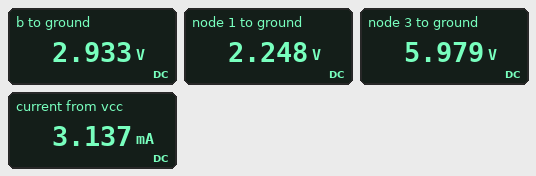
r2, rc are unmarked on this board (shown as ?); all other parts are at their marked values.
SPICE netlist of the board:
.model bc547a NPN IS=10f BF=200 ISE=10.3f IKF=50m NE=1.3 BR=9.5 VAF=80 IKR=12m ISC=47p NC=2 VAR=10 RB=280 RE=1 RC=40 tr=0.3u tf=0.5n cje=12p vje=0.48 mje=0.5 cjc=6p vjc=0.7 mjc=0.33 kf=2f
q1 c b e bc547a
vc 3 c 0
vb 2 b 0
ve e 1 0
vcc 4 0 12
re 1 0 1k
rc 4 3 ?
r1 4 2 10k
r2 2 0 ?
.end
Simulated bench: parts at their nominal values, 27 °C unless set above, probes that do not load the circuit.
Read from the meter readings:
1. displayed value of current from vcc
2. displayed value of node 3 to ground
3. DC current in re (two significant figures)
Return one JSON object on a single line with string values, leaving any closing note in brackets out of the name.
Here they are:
{"displayed value of current from vcc": "3.137 mA", "displayed value of node 3 to ground": "5.979 V", "DC current in re": "2.2 mA"}
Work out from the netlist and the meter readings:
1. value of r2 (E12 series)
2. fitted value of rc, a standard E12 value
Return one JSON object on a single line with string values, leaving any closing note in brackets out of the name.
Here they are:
{"value of r2": "3.3 kΩ", "fitted value of rc, a standard E12 value": "2.7 kΩ"}
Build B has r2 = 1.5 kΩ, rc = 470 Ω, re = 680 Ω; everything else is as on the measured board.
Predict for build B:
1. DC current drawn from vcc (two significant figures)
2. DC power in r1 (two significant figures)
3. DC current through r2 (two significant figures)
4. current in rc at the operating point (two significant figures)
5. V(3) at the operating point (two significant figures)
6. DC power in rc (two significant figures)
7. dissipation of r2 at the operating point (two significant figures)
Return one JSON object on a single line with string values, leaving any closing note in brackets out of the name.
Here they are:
{"DC current drawn from vcc": "2.3 mA", "DC power in r1": "11 mW", "DC current through r2": "1.0 mA", "current in rc at the operating point": "1.3 mA", "V(3) at the operating point": "11 V", "DC power in rc": "790 µW", "dissipation of r2 at the operating point": "1.6 mW"}
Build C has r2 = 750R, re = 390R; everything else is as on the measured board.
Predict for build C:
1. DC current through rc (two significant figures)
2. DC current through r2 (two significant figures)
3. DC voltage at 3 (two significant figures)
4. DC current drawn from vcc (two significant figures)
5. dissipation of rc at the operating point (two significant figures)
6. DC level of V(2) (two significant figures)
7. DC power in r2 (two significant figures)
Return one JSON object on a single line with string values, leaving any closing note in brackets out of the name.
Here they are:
{"DC current through rc": "500 µA", "DC current through r2": "1.1 mA", "DC voltage at 3": "11 V", "DC current drawn from vcc": "1.6 mA", "dissipation of rc at the operating point": "680 µW", "DC level of V(2)": "830 mV", "DC power in r2": "930 µW"}
